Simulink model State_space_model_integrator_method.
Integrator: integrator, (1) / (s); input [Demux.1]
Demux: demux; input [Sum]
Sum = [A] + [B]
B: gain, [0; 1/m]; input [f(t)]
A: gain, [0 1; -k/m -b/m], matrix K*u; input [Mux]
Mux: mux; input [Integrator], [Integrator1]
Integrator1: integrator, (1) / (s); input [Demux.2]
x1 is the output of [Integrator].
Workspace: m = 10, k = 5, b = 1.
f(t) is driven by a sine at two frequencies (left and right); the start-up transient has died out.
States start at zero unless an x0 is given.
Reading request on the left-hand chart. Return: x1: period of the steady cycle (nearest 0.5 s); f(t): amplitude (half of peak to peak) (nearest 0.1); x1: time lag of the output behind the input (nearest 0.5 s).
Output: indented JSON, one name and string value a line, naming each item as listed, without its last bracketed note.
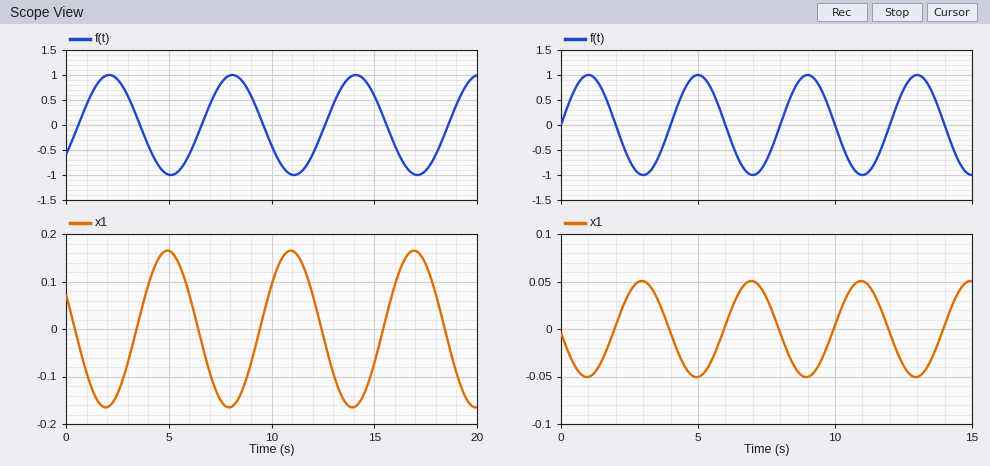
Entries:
{
  "x1: period of the steady cycle": "6.0 s",
  "f(t): amplitude (half of peak to peak)": "1.0",
  "x1: time lag of the output behind the input": "3.0 s"
}
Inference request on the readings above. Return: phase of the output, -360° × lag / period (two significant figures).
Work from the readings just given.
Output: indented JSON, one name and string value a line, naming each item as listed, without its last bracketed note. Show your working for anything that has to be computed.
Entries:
{
  "phase of the output, -360° × lag / period": "-360 × 3 / 6 = -180°"
}
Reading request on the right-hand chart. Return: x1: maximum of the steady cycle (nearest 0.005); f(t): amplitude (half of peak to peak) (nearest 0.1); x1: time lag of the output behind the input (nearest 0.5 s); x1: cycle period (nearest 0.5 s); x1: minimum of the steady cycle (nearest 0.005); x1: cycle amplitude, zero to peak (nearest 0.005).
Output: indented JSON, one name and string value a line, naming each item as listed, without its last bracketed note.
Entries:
{
  "x1: maximum of the steady cycle": "0.050",
  "f(t): amplitude (half of peak to peak)": "1.0",
  "x1: time lag of the output behind the input": "2.0 s",
  "x1: cycle period": "4.0 s",
  "x1: minimum of the steady cycle": "-0.050",
  "x1: cycle amplitude, zero to peak": "0.050"
}
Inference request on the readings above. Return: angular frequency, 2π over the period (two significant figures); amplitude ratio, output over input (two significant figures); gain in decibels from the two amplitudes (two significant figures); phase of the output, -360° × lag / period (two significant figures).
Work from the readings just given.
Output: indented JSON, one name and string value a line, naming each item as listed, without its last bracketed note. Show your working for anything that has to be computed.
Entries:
{
  "angular frequency, 2π over the period": "2π / 4 = 1.6 rad/s",
  "amplitude ratio, output over input": "0.05 / 1 = 0.050",
  "gain in decibels from the two amplitudes": "20 log10(0.05 / 1) = -26 dB",
  "phase of the output, -360° × lag / period": "-360 × 2 / 4 = -180°"
}
